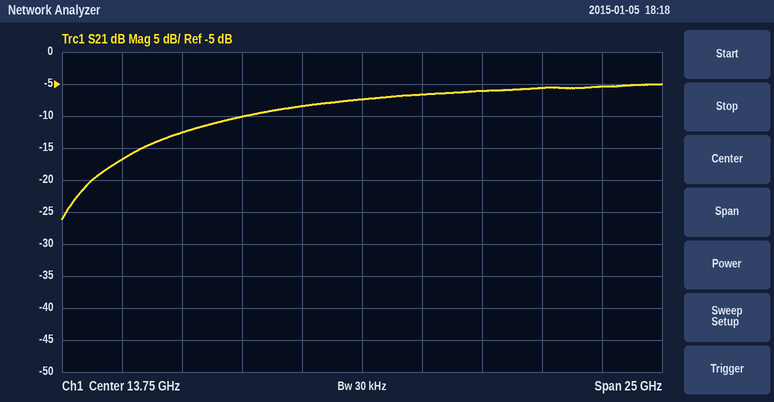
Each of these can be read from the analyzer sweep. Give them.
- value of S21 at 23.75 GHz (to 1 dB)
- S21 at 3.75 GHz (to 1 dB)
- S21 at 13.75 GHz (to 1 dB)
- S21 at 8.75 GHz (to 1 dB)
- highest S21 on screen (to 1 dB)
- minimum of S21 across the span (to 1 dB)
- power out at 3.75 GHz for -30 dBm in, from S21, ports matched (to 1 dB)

-5 dB
-17 dB
-7 dB
-10 dB
-5 dB
-26 dB
-47 dBm
